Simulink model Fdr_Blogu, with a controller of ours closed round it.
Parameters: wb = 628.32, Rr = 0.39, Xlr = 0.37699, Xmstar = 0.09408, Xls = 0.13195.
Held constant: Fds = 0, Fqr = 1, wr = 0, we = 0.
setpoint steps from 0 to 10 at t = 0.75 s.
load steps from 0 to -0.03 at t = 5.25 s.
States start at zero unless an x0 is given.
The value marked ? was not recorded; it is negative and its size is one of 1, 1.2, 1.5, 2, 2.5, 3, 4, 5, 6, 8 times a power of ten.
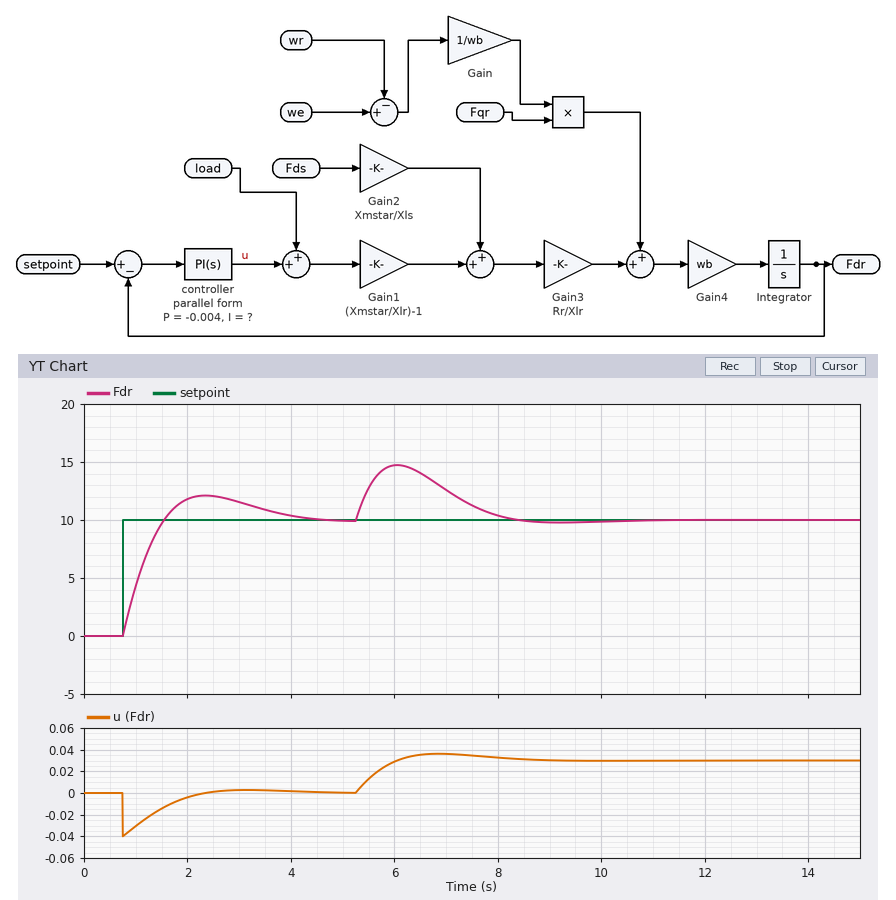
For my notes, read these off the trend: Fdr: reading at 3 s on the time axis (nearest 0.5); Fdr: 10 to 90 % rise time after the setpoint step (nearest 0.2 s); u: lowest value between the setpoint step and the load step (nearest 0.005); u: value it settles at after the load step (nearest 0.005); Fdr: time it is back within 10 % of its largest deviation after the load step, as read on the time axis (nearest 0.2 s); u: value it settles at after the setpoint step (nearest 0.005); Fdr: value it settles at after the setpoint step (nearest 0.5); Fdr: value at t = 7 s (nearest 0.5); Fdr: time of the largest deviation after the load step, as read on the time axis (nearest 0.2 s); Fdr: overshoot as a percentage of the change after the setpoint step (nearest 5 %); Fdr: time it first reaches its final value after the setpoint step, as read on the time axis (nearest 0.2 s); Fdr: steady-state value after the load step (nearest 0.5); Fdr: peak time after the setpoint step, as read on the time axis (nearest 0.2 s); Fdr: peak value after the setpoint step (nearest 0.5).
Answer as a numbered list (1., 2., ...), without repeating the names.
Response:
1. 11.5
2. 0.6 s
3. -0.040
4. 0.030
5. 8.0 s
6. 0.000
7. 10.0
8. 12.5
9. 6.0 s
10. 20 %
11. 1.6 s
12. 10.0
13. 2.4 s
14. 12.0
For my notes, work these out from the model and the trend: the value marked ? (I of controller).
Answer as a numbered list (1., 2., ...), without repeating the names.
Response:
1. -0.004
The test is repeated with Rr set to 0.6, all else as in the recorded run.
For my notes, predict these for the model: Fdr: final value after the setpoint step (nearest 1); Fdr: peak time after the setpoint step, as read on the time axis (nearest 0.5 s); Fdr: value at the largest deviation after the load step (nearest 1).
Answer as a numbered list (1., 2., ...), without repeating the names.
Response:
1. 10
2. 2.0 s
3. 15
